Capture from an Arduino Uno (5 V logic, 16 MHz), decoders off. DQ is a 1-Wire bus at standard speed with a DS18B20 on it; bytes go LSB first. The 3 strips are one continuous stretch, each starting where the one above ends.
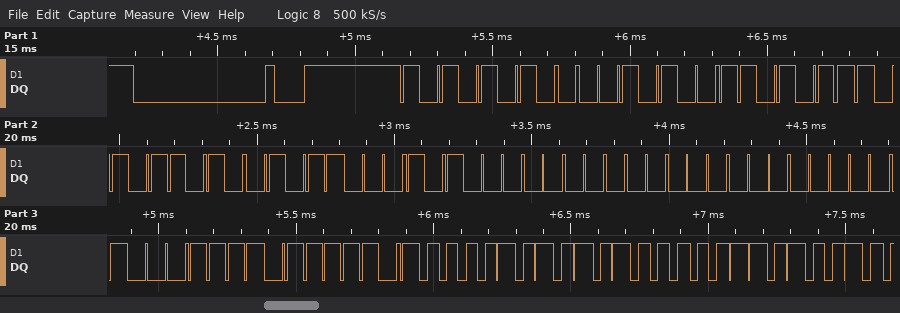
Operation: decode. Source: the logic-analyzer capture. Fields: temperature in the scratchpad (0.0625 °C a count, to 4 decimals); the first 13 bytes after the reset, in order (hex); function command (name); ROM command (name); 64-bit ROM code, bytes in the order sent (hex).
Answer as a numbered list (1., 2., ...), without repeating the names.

1. 85.0000 °C
2. 55 28 EB 5A 1A 05 00 00 F1 BE 50 05 4B
3. Read Scratchpad
4. Match ROM
5. 28 EB 5A 1A 05 00 00 F1
